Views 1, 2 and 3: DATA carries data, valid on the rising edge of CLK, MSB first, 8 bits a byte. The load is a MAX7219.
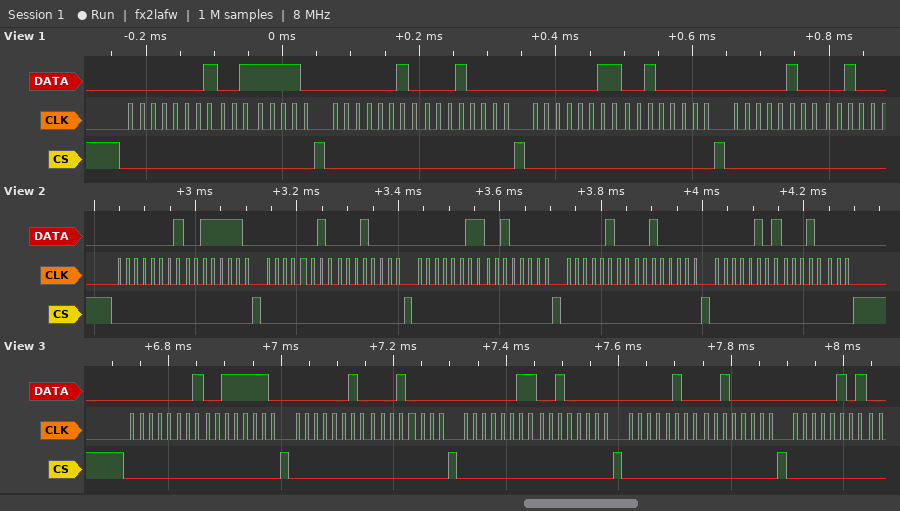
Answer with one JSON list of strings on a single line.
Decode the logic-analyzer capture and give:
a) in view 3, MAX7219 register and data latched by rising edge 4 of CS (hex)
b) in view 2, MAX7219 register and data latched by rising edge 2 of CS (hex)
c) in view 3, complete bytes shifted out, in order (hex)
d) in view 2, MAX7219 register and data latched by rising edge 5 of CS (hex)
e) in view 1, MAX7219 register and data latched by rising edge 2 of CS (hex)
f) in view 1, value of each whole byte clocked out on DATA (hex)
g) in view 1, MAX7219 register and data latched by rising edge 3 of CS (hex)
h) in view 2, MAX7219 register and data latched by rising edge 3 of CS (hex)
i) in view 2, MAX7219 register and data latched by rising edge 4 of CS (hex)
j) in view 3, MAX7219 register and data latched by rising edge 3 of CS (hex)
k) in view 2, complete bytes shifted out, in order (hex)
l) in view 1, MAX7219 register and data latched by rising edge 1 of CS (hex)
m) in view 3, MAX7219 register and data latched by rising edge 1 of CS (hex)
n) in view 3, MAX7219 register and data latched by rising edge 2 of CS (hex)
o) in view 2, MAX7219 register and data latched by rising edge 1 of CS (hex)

["register 0x4, data 0x20", "register 0x2, data 0x10", "0x01 0x3E 0x02 0x10 0x03 0x20 0x04 0x20 0x05", "register 0x5, data 0x10", "register 0x2, data 0x10", "0x01 0x3E 0x02 0x10 0x03 0x20 0x04", "register 0x3, data 0x20", "register 0x3, data 0x20", "register 0x4, data 0x20", "register 0x3, data 0x20", "01 3E 02 10 03 20 04 20 05 10", "register 0x1, data 0x3E", "register 0x1, data 0x3E", "register 0x2, data 0x10", "register 0x1, data 0x3E"]
